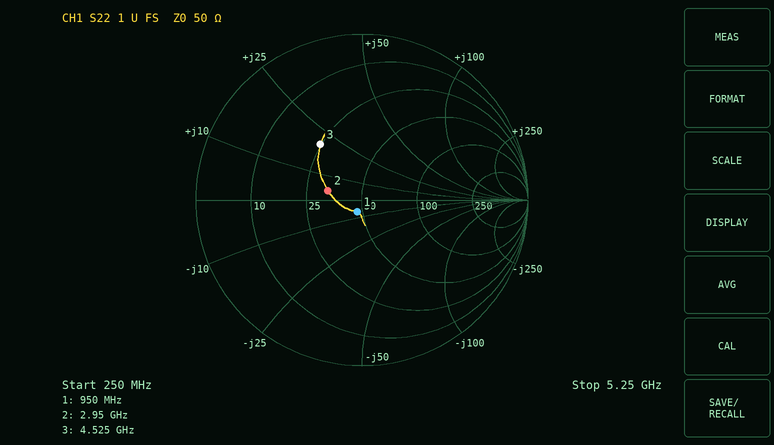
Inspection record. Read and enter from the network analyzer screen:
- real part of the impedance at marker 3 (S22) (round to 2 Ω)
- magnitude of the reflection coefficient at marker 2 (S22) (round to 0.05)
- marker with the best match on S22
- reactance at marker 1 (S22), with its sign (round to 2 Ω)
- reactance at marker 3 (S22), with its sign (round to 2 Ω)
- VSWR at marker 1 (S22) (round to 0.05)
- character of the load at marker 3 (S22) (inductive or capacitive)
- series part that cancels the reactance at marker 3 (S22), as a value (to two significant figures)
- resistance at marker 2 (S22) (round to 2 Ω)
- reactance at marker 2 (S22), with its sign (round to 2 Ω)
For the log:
24 Ω
0.20
marker 1
-6 Ω
+20 Ω
1.15
inductive
1.8 pF
32 Ω
+4 Ω
